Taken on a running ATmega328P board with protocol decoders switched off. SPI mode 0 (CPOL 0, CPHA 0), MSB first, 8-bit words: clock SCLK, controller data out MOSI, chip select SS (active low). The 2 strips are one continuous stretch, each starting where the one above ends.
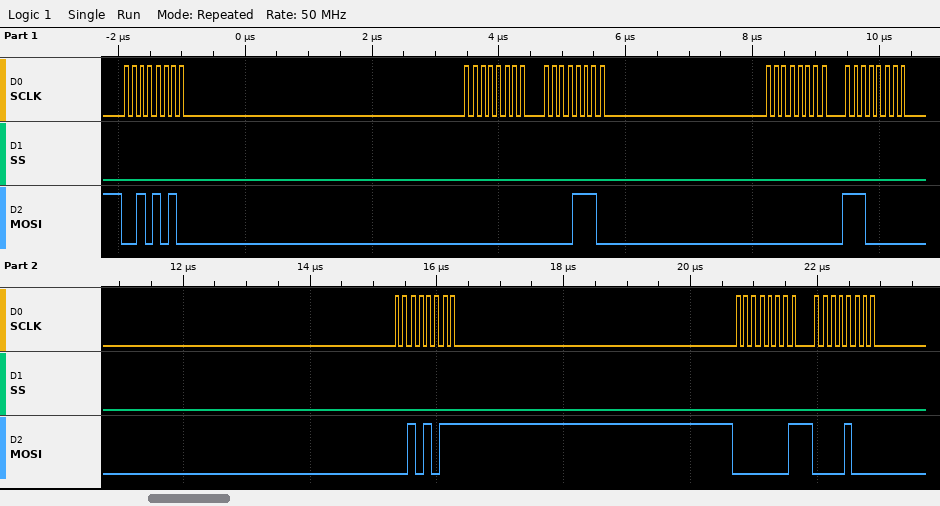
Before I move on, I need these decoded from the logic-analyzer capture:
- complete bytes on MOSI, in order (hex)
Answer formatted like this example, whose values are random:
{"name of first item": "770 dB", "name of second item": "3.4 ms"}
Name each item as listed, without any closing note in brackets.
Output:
{"complete bytes on MOSI, in order": "0x2A 0x00 0x0E 0x00 0xE0 0x2B 0x01 0x08"}
